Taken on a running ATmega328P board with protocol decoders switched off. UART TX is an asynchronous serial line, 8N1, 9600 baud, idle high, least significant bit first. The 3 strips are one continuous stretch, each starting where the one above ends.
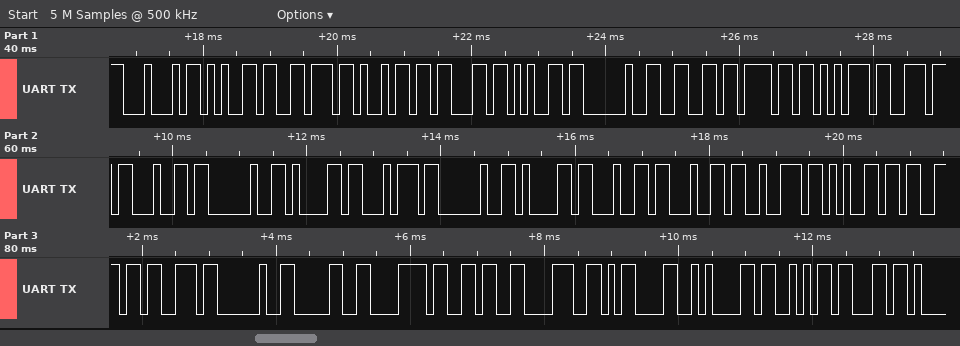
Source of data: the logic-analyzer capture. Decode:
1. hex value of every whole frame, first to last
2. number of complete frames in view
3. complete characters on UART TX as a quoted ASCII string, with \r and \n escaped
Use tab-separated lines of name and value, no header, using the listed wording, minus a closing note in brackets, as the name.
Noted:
hex value of every whole frame, first to last	44 65 76 69 63 65 20 66 6F 75 6E 64 20 61 74 20 61 64 64 72 65 73 73 20 30 78 36 38 0D 0A 53 63
number of complete frames in view	32
complete characters on UART TX as a quoted ASCII string, with \r and \n escaped	"Device found at address 0x68\r\nSc"
